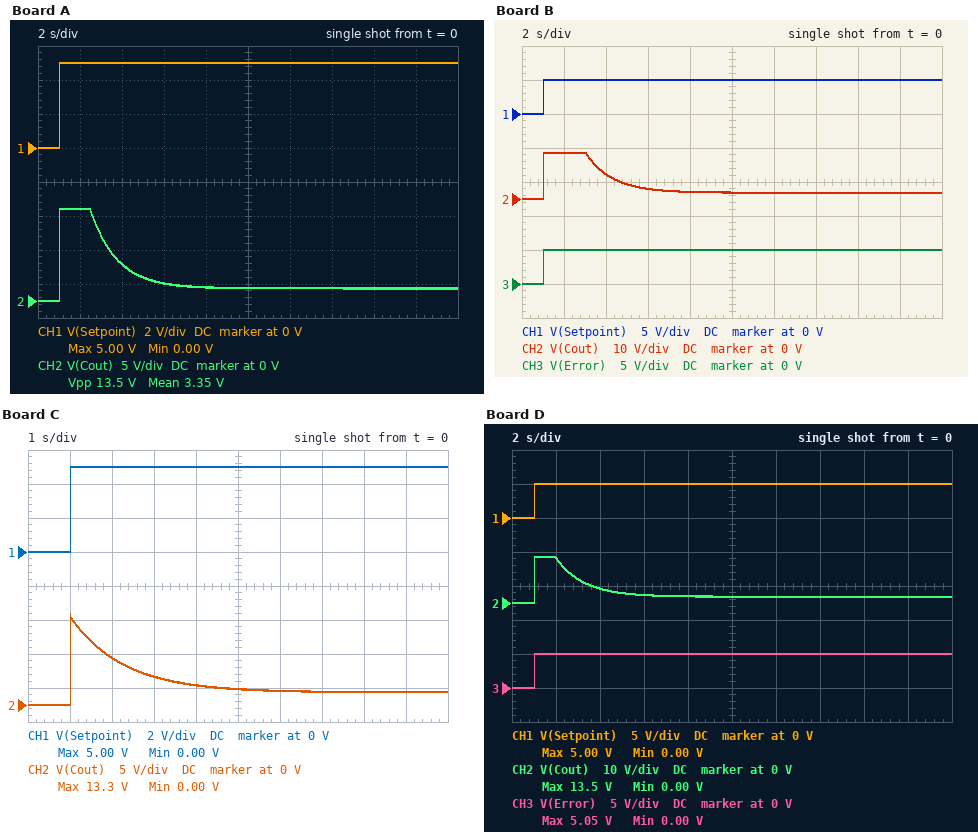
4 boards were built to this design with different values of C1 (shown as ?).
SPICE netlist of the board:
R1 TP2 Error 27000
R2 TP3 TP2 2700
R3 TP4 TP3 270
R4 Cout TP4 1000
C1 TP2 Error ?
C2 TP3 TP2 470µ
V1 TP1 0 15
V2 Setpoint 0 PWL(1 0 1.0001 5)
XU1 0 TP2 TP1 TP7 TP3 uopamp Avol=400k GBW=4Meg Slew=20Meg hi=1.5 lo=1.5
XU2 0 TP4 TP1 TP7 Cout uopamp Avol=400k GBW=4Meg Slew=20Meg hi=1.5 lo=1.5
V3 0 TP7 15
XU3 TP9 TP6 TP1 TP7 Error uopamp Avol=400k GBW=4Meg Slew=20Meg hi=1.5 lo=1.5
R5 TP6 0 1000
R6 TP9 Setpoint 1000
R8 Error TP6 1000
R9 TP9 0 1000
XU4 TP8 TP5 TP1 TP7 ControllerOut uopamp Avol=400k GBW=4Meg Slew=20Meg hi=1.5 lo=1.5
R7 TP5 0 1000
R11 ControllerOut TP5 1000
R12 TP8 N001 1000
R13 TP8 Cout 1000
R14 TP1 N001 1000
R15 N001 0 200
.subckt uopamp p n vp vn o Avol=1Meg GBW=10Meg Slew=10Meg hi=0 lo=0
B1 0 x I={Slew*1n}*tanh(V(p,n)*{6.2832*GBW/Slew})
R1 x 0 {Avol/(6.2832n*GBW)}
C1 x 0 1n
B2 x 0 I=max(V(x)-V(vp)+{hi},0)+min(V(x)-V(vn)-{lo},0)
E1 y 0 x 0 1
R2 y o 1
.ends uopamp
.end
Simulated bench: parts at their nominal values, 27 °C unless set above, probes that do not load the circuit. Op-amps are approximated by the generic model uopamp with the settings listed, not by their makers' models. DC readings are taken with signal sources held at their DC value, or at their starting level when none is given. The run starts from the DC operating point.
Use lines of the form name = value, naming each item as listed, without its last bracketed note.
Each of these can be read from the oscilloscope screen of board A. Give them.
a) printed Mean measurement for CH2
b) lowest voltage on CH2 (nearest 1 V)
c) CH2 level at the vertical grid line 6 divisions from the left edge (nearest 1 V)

printed Mean measurement for CH2 = 3.35 V
lowest voltage on CH2 = 0 V
CH2 level at the vertical grid line 6 divisions from the left edge = 2 V
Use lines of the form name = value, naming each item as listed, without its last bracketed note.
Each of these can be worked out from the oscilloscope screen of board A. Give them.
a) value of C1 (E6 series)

value of C1 = 1 mF
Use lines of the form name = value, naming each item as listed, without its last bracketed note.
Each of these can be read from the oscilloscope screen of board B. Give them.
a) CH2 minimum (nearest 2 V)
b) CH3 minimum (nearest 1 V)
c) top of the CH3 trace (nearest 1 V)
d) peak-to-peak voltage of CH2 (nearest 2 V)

CH2 minimum = 0 V
CH3 minimum = 0 V
top of the CH3 trace = 5 V
peak-to-peak voltage of CH2 = 14 V
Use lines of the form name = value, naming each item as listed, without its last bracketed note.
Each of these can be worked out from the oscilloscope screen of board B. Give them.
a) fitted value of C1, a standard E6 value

fitted value of C1, a standard E6 value = 1.5 mF
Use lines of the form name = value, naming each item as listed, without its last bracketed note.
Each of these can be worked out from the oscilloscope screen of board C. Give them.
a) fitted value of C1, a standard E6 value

fitted value of C1, a standard E6 value = 330 µF
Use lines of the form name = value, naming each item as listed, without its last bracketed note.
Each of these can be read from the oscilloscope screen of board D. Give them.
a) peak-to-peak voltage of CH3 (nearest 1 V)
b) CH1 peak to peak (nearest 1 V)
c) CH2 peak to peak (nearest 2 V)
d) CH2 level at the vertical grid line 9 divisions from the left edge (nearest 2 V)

peak-to-peak voltage of CH3 = 5 V
CH1 peak to peak = 5 V
CH2 peak to peak = 14 V
CH2 level at the vertical grid line 9 divisions from the left edge = 2 V
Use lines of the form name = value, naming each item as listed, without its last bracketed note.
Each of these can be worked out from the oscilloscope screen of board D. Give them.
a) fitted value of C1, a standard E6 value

fitted value of C1, a standard E6 value = 680 µF
